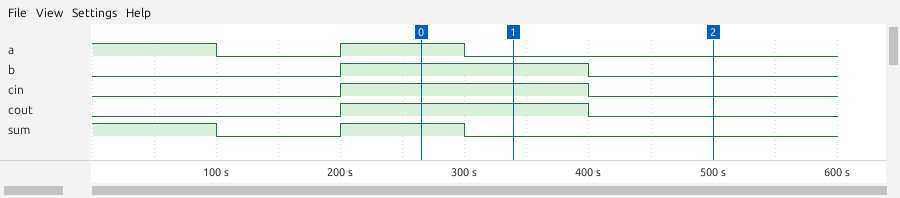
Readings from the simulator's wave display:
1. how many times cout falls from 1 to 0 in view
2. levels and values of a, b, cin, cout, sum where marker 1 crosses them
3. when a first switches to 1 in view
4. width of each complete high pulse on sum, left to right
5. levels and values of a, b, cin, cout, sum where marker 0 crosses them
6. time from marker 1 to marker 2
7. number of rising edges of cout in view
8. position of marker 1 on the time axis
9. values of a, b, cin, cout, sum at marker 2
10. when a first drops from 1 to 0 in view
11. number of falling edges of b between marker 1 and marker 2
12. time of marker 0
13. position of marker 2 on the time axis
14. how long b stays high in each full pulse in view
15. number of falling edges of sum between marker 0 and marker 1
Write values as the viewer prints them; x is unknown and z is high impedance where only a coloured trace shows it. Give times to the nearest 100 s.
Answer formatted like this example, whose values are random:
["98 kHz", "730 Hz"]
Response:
["1", "a=0, b=1, cin=1, cout=1, sum=0", "200 s", "100 s", "a=1, b=1, cin=1, cout=1, sum=1", "200 s", "1", "300 s", "a=0, b=0, cin=0, cout=0, sum=0", "100 s", "1", "300 s", "500 s", "200 s", "1"]
